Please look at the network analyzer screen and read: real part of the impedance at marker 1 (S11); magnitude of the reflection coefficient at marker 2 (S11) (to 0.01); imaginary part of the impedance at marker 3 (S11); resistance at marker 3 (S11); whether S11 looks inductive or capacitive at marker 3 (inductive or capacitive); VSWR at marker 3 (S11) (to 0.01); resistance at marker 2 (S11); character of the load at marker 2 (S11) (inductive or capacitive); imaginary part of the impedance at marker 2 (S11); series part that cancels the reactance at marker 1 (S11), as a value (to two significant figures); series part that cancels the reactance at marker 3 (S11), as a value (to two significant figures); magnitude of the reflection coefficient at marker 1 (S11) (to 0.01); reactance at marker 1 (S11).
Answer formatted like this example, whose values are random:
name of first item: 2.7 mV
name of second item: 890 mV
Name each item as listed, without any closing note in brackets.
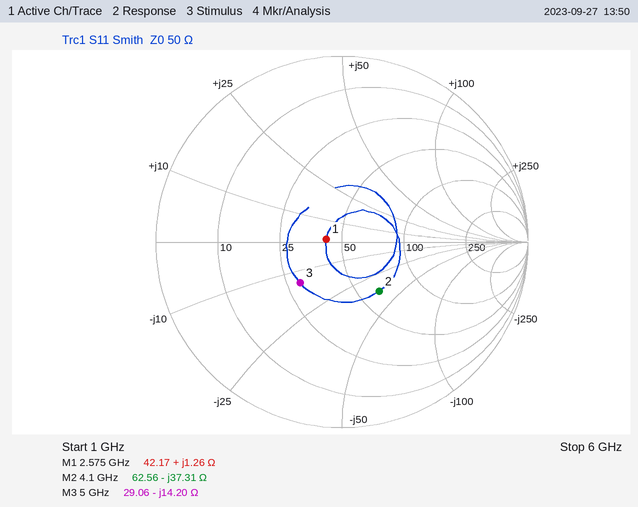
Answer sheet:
real part of the impedance at marker 1: 42.17 Ω
magnitude of the reflection coefficient at marker 2 (S11): 0.33
imaginary part of the impedance at marker 3: -14.20 Ω
resistance at marker 3: 29.06 Ω
whether S11 looks inductive or capacitive at marker 3: capacitive
VSWR at marker 3 (S11): 1.92
resistance at marker 2: 62.56 Ω
character of the load at marker 2 (S11): capacitive
imaginary part of the impedance at marker 2: -37.31 Ω
series part that cancels the reactance at marker 1 (S11), as a value: 49 pF
series part that cancels the reactance at marker 3 (S11), as a value: 450 pH
magnitude of the reflection coefficient at marker 1 (S11): 0.09
reactance at marker 1: +1.26 Ω
